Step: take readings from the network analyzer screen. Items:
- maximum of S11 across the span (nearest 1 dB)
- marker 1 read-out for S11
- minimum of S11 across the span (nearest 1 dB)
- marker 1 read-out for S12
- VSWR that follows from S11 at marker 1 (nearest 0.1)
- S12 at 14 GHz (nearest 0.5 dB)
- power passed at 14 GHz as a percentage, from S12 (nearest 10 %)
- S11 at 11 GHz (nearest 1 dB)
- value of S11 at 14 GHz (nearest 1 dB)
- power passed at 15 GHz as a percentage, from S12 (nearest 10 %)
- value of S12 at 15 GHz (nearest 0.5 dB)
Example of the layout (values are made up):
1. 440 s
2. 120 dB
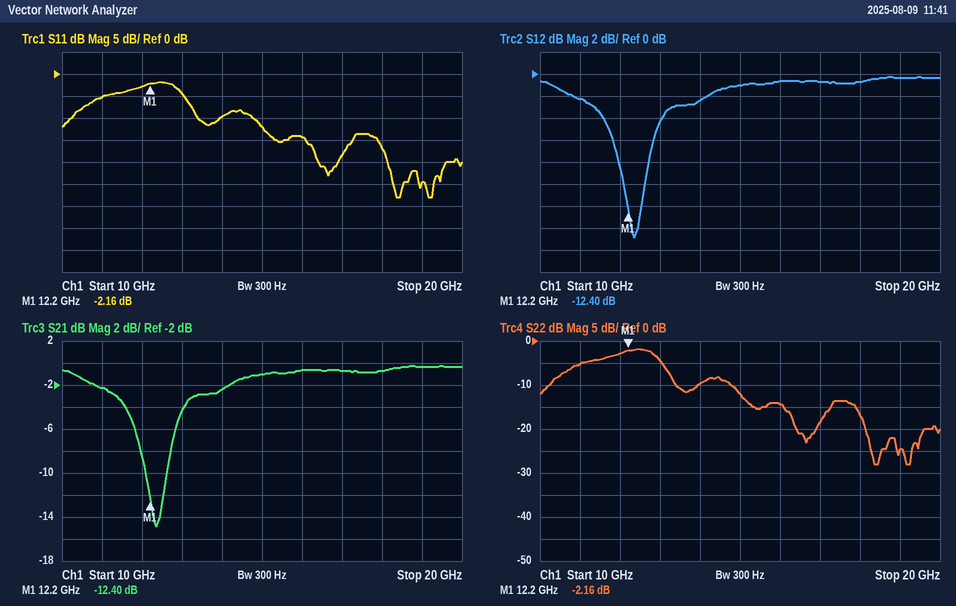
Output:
1. -2 dB
2. -2.16 dB
3. -28 dB
4. -12.40 dB
5. 8.1
6. -2.5 dB
7. 60 %
8. -5 dB
9. -10 dB
10. 80 %
11. -1.0 dB
